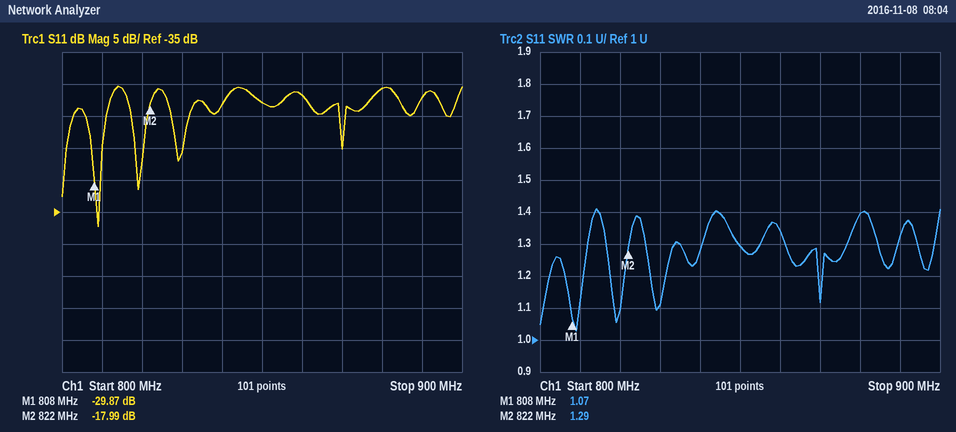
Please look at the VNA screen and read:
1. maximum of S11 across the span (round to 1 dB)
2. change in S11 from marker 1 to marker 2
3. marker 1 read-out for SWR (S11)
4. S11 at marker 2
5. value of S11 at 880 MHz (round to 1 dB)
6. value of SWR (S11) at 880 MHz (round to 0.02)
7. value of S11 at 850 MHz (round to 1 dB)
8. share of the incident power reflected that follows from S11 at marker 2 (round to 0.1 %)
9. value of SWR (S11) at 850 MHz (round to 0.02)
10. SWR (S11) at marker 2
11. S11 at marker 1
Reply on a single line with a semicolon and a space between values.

-15 dB; 11.88 dB; 1.07; -17.99 dB; -16 dB; 1.40; -18 dB; 1.6 %; 1.30; 1.29; -29.87 dB
